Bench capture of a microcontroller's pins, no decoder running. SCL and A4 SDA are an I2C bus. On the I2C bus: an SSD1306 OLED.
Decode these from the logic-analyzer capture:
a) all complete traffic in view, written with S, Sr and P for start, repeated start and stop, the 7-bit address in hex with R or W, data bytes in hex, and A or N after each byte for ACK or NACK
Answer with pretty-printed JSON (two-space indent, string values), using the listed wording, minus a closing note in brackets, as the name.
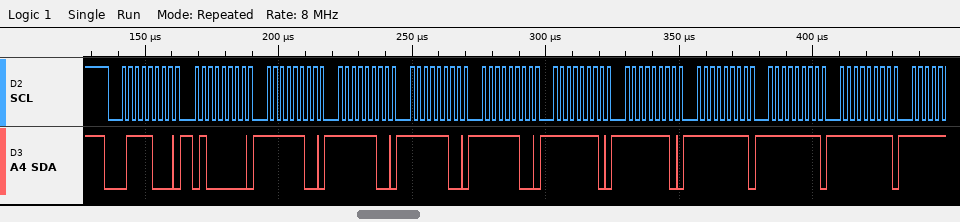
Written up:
{
  "all complete traffic in view, written with S, Sr and P for start, repeated start and stop, the 7-bit address in hex with R or W, data bytes in hex, and A or N after each byte for ACK or NACK": "S 3CW A 40 A FC A FC A FC A FC A FE A FE A FF A FF A FF A"
}
